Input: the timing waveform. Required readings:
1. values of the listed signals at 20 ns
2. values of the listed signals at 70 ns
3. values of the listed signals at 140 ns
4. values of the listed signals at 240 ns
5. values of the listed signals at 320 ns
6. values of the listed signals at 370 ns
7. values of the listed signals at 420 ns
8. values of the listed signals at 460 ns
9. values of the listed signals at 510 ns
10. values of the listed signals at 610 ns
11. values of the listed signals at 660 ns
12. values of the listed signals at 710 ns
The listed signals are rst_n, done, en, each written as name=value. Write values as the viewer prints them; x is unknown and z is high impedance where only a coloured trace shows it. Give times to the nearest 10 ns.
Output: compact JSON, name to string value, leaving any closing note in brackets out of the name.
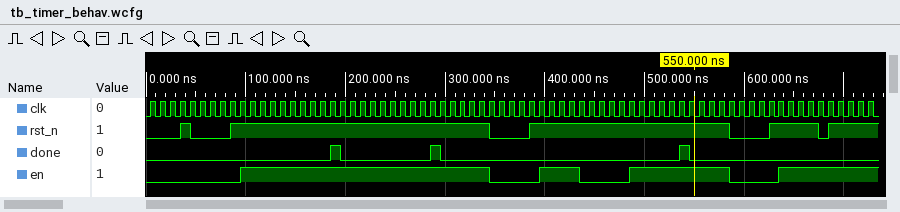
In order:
{"values of the listed signals at 20 ns": "rst_n=0, done=0, en=0", "values of the listed signals at 70 ns": "rst_n=0, done=0, en=0", "values of the listed signals at 140 ns": "rst_n=1, done=0, en=1", "values of the listed signals at 240 ns": "rst_n=1, done=0, en=1", "values of the listed signals at 320 ns": "rst_n=1, done=0, en=1", "values of the listed signals at 370 ns": "rst_n=0, done=0, en=0", "values of the listed signals at 420 ns": "rst_n=1, done=0, en=1", "values of the listed signals at 460 ns": "rst_n=1, done=0, en=0", "values of the listed signals at 510 ns": "rst_n=1, done=0, en=1", "values of the listed signals at 610 ns": "rst_n=0, done=0, en=0", "values of the listed signals at 660 ns": "rst_n=1, done=0, en=1", "values of the listed signals at 710 ns": "rst_n=1, done=0, en=1"}
